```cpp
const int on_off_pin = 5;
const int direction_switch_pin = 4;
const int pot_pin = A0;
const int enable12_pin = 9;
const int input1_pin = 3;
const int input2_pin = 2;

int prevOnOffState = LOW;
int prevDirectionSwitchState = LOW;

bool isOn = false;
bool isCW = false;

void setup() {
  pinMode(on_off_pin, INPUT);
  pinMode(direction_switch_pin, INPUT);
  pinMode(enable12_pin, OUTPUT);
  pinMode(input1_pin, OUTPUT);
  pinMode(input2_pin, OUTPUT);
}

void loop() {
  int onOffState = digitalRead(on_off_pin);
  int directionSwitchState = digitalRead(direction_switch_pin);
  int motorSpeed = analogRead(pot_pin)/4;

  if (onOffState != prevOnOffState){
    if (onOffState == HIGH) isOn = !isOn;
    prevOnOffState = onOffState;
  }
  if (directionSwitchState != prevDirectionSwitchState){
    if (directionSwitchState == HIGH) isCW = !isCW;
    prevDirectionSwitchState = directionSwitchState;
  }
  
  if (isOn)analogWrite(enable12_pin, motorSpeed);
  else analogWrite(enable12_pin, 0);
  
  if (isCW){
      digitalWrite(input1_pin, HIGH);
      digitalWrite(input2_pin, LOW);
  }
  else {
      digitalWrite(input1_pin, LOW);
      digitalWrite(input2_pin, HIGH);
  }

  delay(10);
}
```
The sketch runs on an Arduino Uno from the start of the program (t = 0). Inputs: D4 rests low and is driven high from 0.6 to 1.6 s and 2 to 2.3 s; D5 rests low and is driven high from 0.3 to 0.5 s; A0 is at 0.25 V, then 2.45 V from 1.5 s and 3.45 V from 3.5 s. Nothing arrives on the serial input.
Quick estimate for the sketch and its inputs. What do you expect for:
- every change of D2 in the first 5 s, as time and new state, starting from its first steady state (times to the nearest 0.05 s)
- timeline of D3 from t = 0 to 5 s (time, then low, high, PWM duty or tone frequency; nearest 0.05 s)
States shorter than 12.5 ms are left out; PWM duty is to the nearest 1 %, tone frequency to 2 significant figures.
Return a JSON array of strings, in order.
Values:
["0 s high; 0.6 s low; 2 s high", "0 s low; 0.6 s high; 2 s low"]
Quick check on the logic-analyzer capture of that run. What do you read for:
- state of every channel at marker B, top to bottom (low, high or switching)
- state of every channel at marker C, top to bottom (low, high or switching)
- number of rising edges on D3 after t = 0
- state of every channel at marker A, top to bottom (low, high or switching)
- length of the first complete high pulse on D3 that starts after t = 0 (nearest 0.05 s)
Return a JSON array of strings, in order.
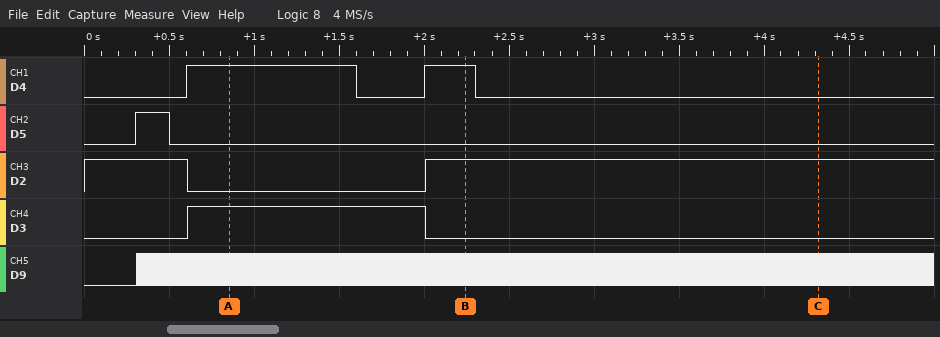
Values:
["D4 high, D5 low, D2 high, D3 low, D9 switching", "D4 low, D5 low, D2 high, D3 low, D9 switching", "1", "D4 high, D5 low, D2 low, D3 high, D9 switching", "1.40 s"]
